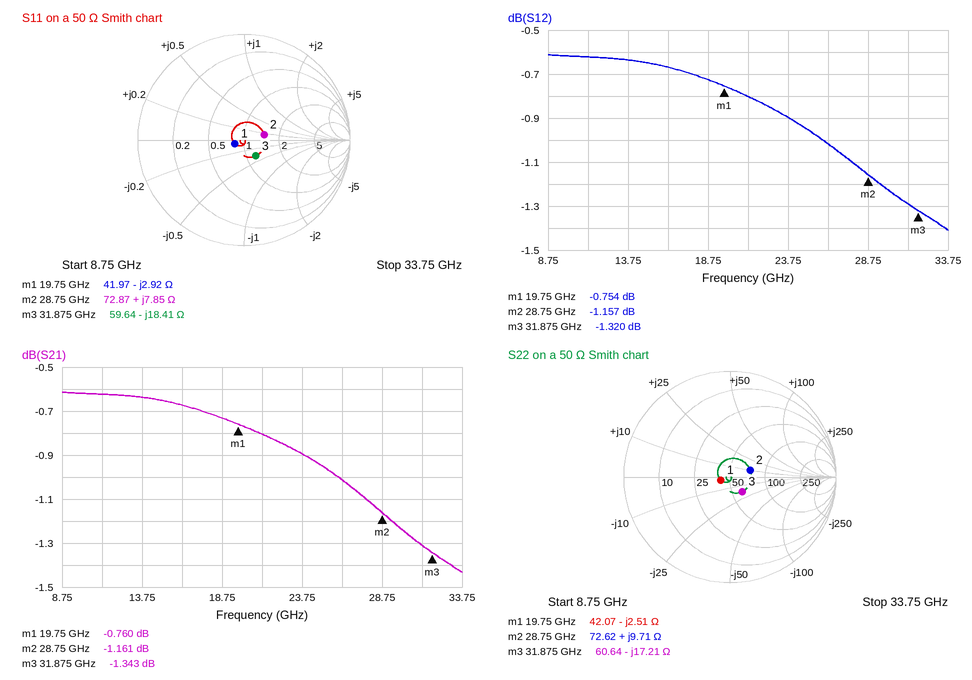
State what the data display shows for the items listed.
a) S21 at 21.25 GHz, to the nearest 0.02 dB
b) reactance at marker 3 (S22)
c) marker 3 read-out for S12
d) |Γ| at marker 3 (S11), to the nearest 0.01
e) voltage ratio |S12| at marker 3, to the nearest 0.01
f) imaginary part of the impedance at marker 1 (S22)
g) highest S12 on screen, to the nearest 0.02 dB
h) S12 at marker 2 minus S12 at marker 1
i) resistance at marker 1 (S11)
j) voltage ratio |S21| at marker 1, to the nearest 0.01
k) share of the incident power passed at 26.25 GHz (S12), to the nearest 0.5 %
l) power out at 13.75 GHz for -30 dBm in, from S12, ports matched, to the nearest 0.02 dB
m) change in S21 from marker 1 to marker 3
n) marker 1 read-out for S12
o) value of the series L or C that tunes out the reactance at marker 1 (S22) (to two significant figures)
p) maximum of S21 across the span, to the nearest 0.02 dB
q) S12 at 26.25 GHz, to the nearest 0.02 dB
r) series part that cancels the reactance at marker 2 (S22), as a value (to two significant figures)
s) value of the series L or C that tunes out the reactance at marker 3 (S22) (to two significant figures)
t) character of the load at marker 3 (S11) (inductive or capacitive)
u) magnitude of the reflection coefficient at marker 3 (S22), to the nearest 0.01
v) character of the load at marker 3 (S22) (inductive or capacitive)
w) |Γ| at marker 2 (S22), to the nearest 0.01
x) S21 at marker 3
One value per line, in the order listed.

-0.80 dB
-17.21 Ω
-1.320 dB
0.19
0.86
-2.51 Ω
-0.62 dB
-0.403 dB
41.97 Ω
0.92
79.0 %
-30.64 dBm
-0.583 dB
-0.754 dB
20 pH
-0.62 dB
-1.02 dB
570 fF
86 pH
capacitive
0.18
capacitive
0.20
-1.343 dB
